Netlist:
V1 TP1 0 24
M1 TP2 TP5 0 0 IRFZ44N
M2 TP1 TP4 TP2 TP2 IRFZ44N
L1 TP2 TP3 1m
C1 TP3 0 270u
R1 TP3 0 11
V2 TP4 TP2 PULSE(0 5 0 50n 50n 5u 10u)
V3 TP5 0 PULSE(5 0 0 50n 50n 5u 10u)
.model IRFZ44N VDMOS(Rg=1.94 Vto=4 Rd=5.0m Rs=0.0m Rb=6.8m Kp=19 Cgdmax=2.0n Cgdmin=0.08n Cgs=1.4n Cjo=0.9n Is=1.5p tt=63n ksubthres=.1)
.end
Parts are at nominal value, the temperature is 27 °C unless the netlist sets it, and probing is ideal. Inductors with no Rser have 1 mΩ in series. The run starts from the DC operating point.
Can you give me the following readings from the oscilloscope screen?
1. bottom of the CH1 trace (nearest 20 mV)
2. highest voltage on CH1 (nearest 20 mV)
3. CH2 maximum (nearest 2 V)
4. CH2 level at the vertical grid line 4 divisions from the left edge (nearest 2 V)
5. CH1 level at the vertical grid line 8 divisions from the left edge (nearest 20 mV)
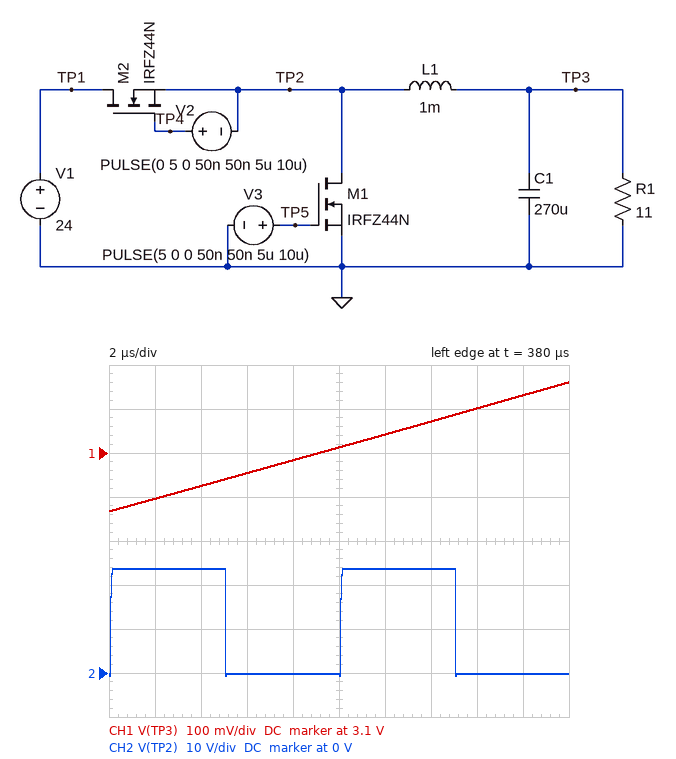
2.96 V
3.26 V
24 V
0 V
3.20 V
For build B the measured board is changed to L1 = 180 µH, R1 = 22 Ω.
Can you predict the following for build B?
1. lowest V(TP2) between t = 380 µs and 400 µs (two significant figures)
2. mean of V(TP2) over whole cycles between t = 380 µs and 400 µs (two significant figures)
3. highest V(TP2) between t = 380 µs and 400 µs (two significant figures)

-800 mV
10 V
23 V
